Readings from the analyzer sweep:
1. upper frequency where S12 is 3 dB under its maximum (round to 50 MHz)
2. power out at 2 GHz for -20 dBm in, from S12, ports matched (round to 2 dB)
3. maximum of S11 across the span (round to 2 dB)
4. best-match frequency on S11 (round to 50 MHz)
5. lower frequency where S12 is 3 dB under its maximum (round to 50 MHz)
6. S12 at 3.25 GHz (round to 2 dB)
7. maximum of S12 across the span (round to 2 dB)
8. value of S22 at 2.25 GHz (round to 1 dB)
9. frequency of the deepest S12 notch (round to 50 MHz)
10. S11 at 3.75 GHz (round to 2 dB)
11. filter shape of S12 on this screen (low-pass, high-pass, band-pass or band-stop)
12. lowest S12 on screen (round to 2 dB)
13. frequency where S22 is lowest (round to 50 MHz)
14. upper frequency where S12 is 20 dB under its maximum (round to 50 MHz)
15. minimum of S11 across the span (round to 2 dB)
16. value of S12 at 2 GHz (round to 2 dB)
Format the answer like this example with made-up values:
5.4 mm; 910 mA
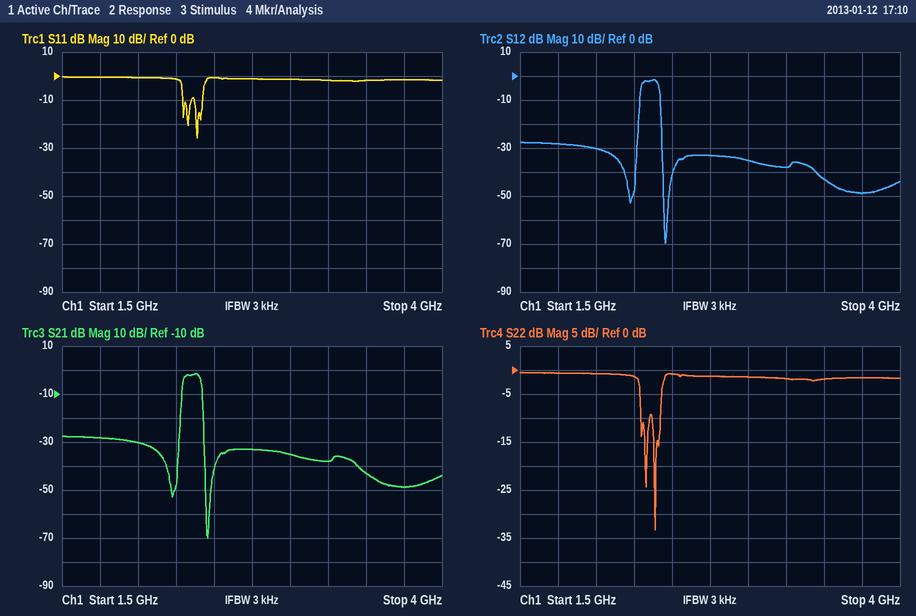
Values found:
2.40 GHz; -50 dBm; 0 dB; 2.40 GHz; 2.30 GHz; -38 dB; -2 dB; -1 dB; 2.45 GHz; -2 dB; band-pass; -70 dB; 2.40 GHz; 2.45 GHz; -26 dB; -30 dB
